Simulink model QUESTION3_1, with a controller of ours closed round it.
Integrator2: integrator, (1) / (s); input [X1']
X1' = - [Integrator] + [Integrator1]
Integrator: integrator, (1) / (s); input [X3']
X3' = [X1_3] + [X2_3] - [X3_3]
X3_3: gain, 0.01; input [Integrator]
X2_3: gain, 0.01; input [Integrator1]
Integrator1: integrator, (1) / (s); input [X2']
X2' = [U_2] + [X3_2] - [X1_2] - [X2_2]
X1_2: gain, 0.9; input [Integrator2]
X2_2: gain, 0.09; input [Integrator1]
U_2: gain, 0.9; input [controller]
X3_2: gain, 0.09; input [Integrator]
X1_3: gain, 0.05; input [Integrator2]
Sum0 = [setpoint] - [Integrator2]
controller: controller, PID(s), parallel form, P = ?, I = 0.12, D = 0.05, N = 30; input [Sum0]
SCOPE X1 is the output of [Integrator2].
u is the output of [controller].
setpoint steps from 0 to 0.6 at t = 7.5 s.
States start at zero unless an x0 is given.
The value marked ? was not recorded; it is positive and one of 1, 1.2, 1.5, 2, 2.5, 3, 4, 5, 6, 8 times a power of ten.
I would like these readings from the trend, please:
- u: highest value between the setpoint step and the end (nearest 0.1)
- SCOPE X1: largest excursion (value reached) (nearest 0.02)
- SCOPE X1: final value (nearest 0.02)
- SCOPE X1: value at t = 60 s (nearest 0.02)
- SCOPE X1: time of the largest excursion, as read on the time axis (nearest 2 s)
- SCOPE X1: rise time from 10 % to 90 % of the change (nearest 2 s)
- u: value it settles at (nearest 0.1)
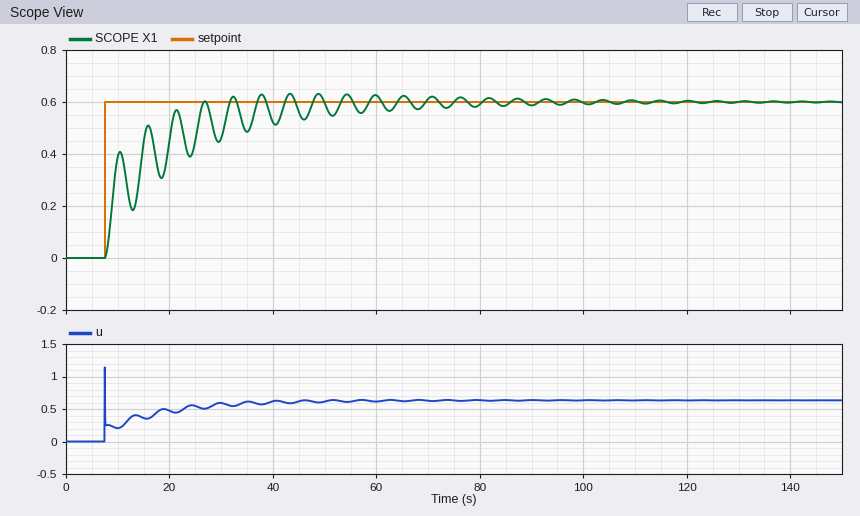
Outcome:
1.1
0.64
0.60
0.62
44 s
12 s
0.6
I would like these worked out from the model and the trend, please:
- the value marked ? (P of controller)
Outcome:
0.4
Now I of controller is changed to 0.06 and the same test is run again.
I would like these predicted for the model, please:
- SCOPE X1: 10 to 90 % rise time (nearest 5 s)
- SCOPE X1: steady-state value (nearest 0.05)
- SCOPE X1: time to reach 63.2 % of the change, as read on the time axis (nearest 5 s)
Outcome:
40 s
0.60
15 s
